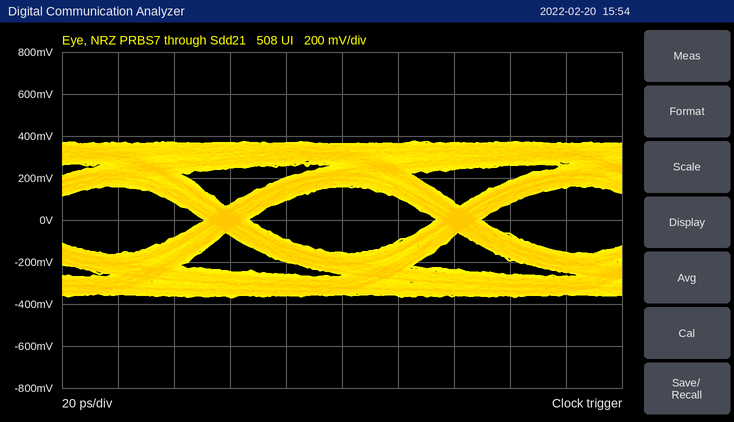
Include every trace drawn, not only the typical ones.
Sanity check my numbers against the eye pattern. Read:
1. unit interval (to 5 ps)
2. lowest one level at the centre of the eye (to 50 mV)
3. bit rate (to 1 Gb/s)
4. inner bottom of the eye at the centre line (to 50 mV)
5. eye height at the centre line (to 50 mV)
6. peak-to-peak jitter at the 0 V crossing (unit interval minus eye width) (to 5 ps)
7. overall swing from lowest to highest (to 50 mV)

85 ps
150 mV
12 Gb/s
-150 mV
300 mV
15 ps
750 mV
